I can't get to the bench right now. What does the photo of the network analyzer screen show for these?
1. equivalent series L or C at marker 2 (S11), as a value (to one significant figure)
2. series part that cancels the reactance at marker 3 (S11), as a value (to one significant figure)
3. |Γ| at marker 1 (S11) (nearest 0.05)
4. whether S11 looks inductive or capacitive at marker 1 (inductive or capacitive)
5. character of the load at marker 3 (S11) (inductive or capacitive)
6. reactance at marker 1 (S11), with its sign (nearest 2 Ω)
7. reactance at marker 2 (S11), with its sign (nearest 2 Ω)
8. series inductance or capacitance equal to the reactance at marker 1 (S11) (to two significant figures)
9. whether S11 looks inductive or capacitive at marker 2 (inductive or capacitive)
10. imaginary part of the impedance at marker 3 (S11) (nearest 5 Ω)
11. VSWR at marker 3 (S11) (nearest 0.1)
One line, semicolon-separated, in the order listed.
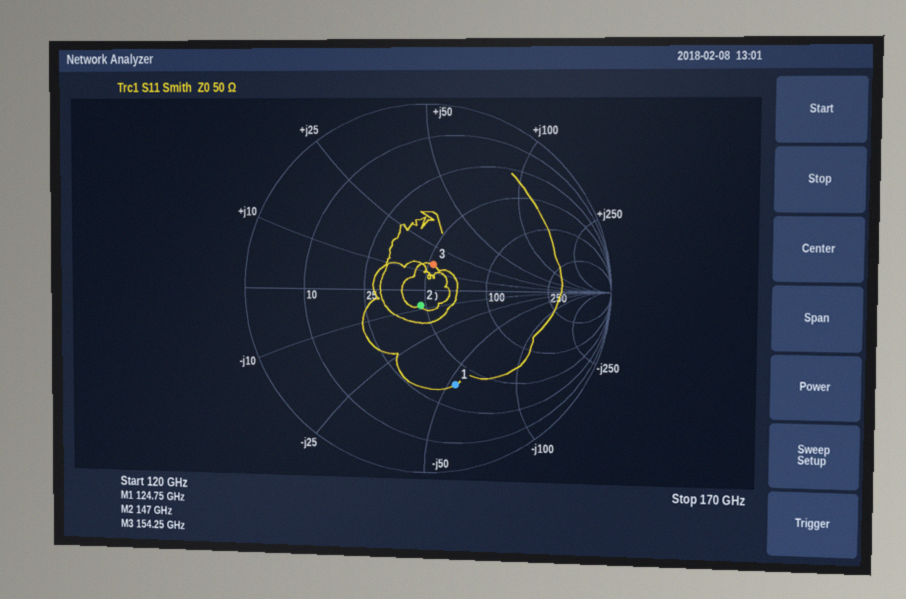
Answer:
100 fF; 70 fF; 0.55; capacitive; inductive; -54 Ω; -8 Ω; 24 fF; capacitive; +15 Ω; 1.3
